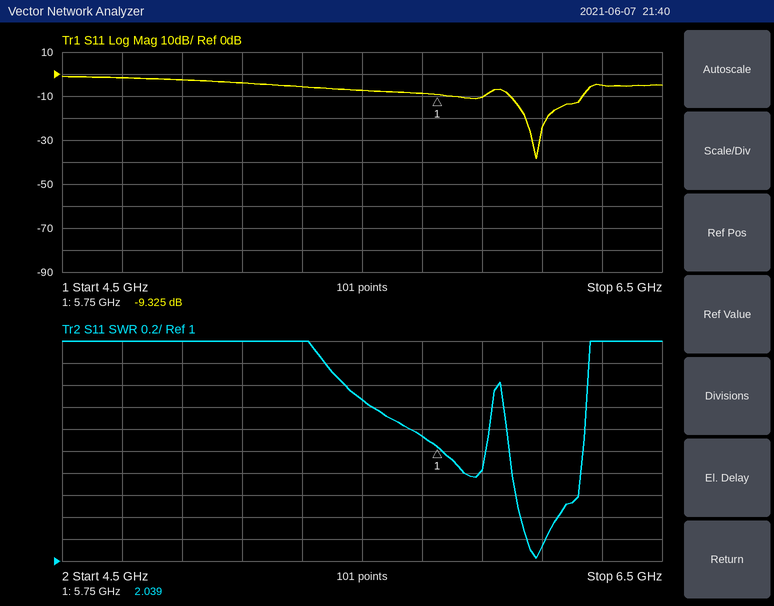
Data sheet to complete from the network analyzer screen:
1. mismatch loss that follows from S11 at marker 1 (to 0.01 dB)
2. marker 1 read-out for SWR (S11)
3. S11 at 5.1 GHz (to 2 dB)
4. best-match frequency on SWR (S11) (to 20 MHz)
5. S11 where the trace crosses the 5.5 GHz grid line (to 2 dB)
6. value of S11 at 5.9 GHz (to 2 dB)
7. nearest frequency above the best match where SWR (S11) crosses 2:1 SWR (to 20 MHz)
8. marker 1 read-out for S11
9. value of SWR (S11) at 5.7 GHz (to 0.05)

0.54 dB
2.039
-4 dB
6.08 GHz
-8 dB
-10 dB
6.24 GHz
-9.325 dB
2.15
